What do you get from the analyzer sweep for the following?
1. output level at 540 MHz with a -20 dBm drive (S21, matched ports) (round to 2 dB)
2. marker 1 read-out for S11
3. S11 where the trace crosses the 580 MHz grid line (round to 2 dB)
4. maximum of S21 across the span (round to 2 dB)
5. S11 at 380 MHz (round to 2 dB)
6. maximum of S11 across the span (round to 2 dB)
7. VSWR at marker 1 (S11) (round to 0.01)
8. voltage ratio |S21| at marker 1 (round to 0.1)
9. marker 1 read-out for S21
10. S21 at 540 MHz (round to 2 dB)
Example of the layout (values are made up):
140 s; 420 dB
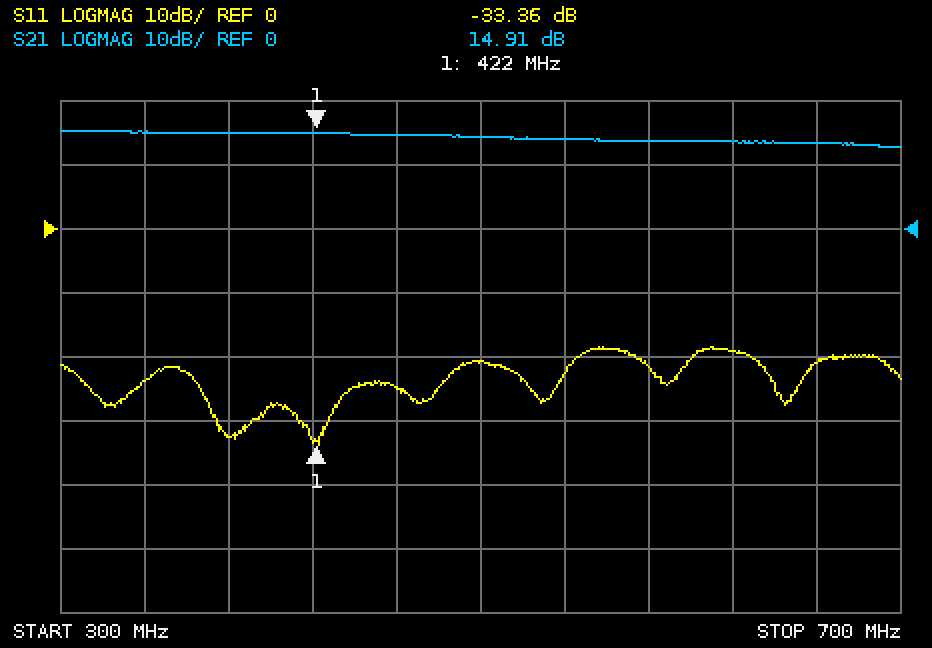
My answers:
-6 dBm; -33.36 dB; -22 dB; 16 dB; -32 dB; -18 dB; 1.04; 5.6; 14.91 dB; 14 dB
